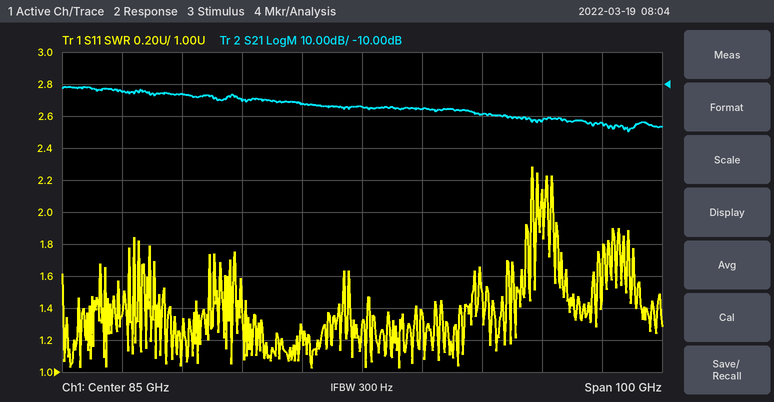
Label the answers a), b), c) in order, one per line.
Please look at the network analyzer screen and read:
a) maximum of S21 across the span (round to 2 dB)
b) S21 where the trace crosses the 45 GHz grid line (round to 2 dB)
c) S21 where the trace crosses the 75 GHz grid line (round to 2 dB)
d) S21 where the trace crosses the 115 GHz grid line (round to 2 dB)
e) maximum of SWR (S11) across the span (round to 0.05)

a) -10 dB
b) -12 dB
c) -16 dB
d) -22 dB
e) 2.30
